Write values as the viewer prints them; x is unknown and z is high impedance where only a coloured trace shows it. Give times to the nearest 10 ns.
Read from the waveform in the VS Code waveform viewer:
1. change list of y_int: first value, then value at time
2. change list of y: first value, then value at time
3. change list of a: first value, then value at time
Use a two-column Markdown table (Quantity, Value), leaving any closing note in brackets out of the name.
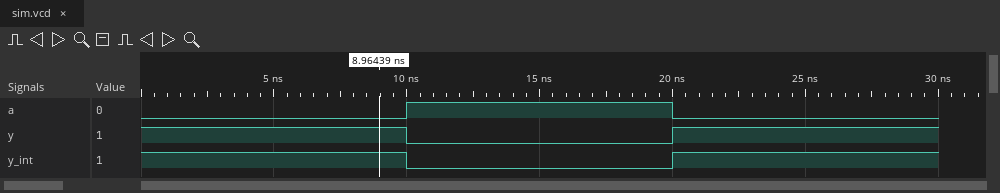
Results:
| Quantity | Value |
|---|---|
| change list of y_int: first value, then value at time | 1, 0 at 10 ns, 1 at 20 ns |
| change list of y: first value, then value at time | 1, 0 at 10 ns, 1 at 20 ns |
| change list of a: first value, then value at time | 0, 1 at 10 ns, 0 at 20 ns |
